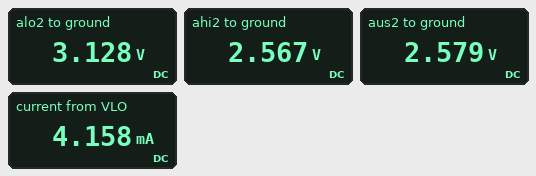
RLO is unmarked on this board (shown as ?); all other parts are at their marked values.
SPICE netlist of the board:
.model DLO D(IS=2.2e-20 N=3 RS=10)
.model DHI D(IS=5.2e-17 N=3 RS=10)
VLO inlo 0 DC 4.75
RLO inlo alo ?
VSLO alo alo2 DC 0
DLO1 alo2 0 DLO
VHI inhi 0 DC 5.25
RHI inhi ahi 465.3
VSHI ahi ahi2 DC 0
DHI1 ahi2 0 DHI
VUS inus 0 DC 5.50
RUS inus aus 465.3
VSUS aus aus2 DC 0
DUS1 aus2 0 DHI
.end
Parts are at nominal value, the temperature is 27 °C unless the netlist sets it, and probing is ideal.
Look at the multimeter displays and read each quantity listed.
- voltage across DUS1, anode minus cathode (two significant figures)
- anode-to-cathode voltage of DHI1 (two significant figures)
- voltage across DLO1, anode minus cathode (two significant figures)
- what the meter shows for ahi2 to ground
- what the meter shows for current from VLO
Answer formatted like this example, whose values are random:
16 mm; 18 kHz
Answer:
2.6 V; 2.6 V; 3.1 V; 2.567 V; 4.158 mA
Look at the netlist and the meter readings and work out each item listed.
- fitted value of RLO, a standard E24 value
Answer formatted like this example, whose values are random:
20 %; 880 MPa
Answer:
390 Ω
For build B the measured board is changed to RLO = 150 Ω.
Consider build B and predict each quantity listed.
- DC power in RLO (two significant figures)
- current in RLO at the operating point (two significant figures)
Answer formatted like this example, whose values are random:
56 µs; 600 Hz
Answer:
15 mW; 10 mA
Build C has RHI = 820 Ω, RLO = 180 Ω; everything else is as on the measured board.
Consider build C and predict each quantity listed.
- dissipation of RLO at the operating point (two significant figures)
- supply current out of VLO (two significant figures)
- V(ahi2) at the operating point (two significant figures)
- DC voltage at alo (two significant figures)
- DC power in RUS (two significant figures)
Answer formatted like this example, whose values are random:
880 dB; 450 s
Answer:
13 mW; 8.5 mA; 2.5 V; 3.2 V; 18 mW
